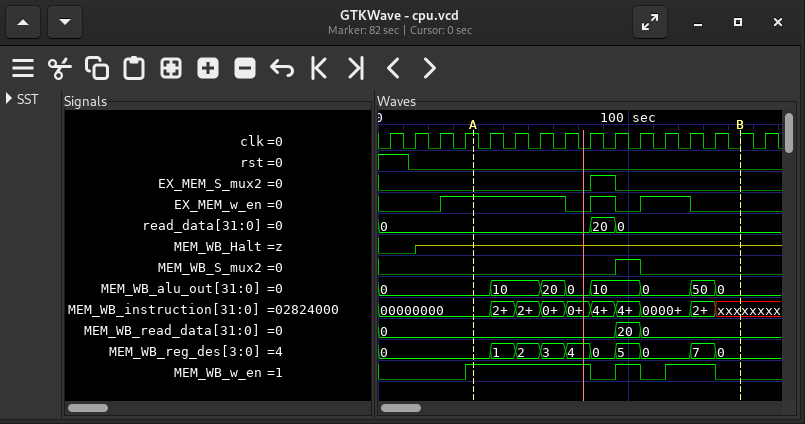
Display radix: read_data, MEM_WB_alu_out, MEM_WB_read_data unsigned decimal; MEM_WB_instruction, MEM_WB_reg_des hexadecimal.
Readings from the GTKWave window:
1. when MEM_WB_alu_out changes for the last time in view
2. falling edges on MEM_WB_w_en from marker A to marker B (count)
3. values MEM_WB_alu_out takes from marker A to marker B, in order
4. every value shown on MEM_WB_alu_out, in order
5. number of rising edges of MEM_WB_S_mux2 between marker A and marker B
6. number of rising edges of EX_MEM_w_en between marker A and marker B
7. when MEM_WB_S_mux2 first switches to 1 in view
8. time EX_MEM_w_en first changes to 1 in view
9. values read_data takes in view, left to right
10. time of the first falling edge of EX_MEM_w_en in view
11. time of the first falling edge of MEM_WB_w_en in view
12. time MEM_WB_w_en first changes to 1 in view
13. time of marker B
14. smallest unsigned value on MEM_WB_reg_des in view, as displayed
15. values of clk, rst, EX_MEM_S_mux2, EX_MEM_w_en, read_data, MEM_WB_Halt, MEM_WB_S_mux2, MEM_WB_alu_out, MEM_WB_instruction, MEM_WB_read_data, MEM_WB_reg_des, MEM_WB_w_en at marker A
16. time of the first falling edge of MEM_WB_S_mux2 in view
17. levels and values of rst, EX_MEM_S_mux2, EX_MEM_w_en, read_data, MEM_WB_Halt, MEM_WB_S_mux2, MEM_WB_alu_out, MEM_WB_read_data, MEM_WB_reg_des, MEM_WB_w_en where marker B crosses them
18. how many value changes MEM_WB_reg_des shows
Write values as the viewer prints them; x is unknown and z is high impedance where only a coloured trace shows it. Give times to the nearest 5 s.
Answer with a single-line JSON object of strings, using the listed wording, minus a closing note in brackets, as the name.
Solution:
{"when MEM_WB_alu_out changes for the last time in view": "135 s", "falling edges on MEM_WB_w_en from marker A to marker B": "3", "values MEM_WB_alu_out takes from marker A to marker B, in order": "0, 10, 20, 0, 10, 0, 50, 0", "every value shown on MEM_WB_alu_out, in order": "0, 10, 20, 0, 10, 0, 50, 0", "number of rising edges of MEM_WB_S_mux2 between marker A and marker B": "1", "number of rising edges of EX_MEM_w_en between marker A and marker B": "2", "when MEM_WB_S_mux2 first switches to 1 in view": "95 s", "time EX_MEM_w_en first changes to 1 in view": "25 s", "values read_data takes in view, left to right": "0, 20, 0", "time of the first falling edge of EX_MEM_w_en in view": "75 s", "time of the first falling edge of MEM_WB_w_en in view": "85 s", "time MEM_WB_w_en first changes to 1 in view": "35 s", "time of marker B": "145 s", "smallest unsigned value on MEM_WB_reg_des in view, as displayed": "0", "values of clk, rst, EX_MEM_S_mux2, EX_MEM_w_en, read_data, MEM_WB_Halt, MEM_WB_S_mux2, MEM_WB_alu_out, MEM_WB_instruction, MEM_WB_read_data, MEM_WB_reg_des, MEM_WB_w_en at marker A": "clk=1, rst=0, EX_MEM_S_mux2=0, EX_MEM_w_en=1, read_data=0, MEM_WB_Halt=z, MEM_WB_S_mux2=0, MEM_WB_alu_out=0, MEM_WB_instruction=00000000, MEM_WB_read_data=0, MEM_WB_reg_des=0, MEM_WB_w_en=1", "time of the first falling edge of MEM_WB_S_mux2 in view": "105 s", "levels and values of rst, EX_MEM_S_mux2, EX_MEM_w_en, read_data, MEM_WB_Halt, MEM_WB_S_mux2, MEM_WB_alu_out, MEM_WB_read_data, MEM_WB_reg_des, MEM_WB_w_en where marker B crosses them": "rst=0, EX_MEM_S_mux2=0, EX_MEM_w_en=0, read_data=0, MEM_WB_Halt=z, MEM_WB_S_mux2=0, MEM_WB_alu_out=0, MEM_WB_read_data=0, MEM_WB_reg_des=0, MEM_WB_w_en=0", "how many value changes MEM_WB_reg_des shows": "9"}
